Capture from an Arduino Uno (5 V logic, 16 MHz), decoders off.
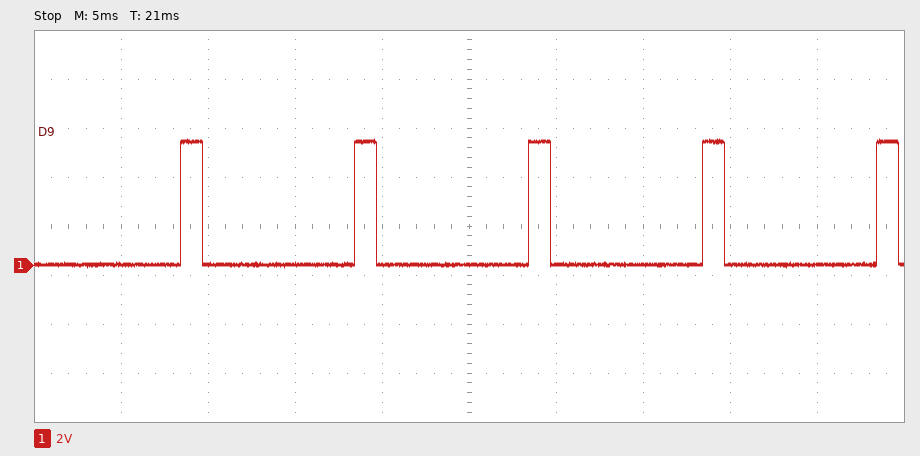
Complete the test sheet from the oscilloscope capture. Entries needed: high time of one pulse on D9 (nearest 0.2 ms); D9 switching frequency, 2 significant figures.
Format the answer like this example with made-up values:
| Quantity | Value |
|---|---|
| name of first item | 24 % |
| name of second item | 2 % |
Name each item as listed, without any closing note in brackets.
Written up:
| Quantity | Value |
|---|---|
| high time of one pulse on D9 | 1.2 ms |
| D9 switching frequency, 2 significant figures | 100 Hz |
